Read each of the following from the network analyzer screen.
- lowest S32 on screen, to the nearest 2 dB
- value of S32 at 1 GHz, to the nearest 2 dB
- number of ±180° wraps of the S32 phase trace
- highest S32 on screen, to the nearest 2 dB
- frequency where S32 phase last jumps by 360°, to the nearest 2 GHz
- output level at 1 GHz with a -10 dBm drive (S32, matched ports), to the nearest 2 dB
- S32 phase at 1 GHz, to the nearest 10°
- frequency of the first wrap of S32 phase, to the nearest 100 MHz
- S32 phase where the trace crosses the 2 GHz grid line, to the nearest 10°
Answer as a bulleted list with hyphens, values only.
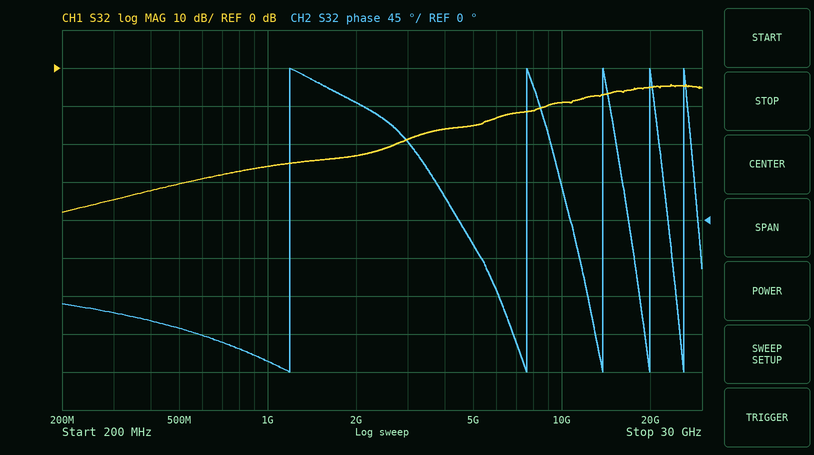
- -38 dB
- -26 dB
- 5
- -4 dB
- 26 GHz
- -36 dBm
- -170°
- 1.2 GHz
- 140°
